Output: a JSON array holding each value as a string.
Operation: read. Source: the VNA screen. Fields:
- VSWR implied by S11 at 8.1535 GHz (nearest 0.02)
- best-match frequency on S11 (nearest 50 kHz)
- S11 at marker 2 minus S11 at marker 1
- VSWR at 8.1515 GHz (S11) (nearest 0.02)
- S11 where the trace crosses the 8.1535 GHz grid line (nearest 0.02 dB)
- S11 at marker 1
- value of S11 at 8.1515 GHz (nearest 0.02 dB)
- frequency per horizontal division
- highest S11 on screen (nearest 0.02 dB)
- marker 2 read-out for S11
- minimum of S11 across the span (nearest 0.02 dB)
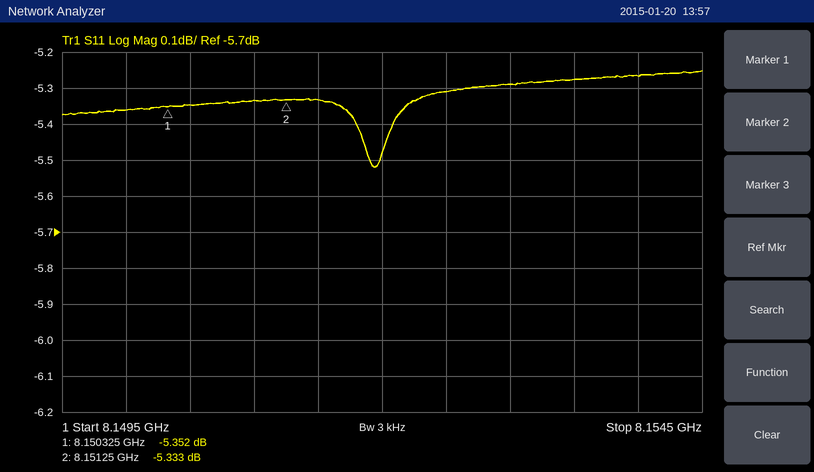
["3.40", "8.15195 GHz", "0.019 dB", "3.36", "-5.28 dB", "-5.352 dB", "-5.34 dB", "500 kHz", "-5.26 dB", "-5.333 dB", "-5.52 dB"]
